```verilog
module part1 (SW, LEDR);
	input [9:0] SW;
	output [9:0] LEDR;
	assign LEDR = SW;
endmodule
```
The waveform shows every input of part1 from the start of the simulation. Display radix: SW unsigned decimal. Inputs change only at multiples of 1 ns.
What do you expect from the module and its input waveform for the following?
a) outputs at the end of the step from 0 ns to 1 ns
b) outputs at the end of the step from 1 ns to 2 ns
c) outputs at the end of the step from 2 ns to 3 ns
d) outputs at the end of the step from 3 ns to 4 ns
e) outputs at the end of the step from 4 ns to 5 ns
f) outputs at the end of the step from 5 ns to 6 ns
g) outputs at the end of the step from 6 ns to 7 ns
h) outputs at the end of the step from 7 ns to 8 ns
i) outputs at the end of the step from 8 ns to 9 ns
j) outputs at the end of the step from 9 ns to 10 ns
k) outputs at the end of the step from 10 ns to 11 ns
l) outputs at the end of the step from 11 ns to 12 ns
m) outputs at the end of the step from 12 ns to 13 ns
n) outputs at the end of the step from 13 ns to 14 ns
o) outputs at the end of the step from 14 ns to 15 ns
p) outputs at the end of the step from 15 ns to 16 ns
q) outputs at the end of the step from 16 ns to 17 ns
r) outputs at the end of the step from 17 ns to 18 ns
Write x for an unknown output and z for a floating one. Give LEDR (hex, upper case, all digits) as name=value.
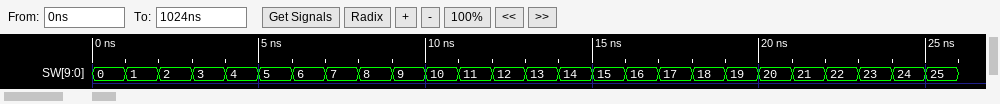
LEDR=000
LEDR=001
LEDR=002
LEDR=003
LEDR=004
LEDR=005
LEDR=006
LEDR=007
LEDR=008
LEDR=009
LEDR=00A
LEDR=00B
LEDR=00C
LEDR=00D
LEDR=00E
LEDR=00F
LEDR=010
LEDR=011
